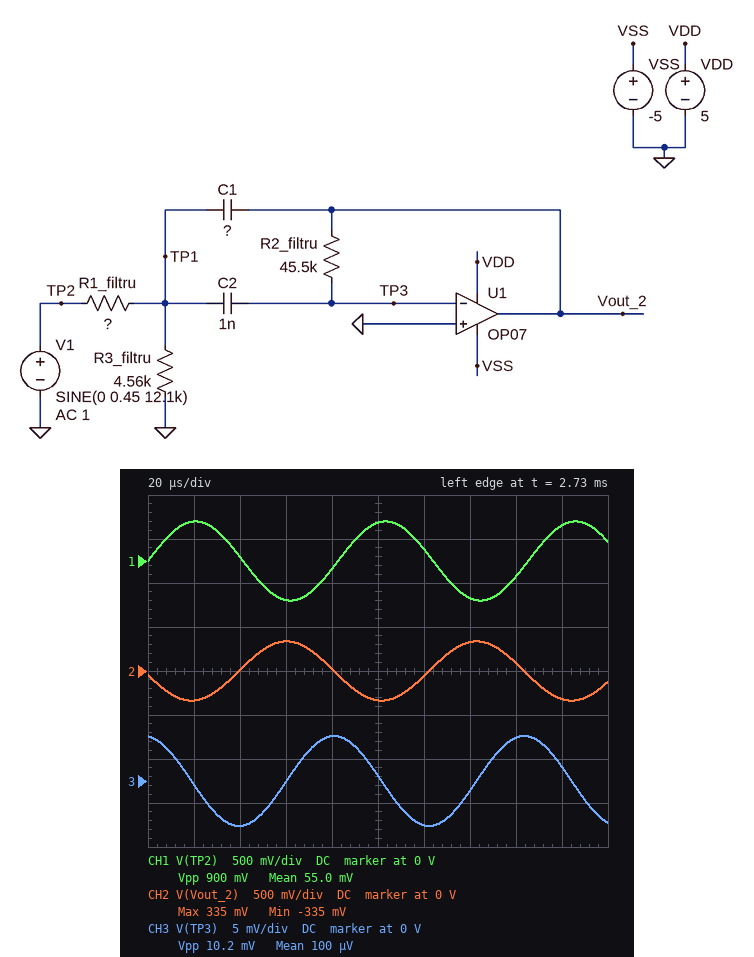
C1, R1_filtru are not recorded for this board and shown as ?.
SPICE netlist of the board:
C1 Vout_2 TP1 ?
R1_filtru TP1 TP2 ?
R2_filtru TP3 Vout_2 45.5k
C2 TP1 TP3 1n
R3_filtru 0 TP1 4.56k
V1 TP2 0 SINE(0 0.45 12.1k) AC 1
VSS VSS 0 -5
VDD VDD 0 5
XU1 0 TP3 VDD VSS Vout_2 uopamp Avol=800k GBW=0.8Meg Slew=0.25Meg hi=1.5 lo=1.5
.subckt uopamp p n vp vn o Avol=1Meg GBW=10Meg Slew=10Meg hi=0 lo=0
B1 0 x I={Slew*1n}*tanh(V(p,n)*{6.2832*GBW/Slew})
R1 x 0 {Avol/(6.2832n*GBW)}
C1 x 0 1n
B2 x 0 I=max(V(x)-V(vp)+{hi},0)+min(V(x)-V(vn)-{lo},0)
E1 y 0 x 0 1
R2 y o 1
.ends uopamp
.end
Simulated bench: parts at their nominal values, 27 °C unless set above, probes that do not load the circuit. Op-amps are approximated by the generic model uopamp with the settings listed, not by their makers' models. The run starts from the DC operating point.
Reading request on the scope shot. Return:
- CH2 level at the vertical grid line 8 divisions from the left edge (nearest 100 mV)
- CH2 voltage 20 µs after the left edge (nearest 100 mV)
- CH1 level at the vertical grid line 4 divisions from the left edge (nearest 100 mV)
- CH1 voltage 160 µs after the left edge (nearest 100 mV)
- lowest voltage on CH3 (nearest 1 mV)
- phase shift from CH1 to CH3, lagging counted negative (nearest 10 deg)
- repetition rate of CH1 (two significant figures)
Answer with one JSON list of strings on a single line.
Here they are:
["100 mV", "-300 mV", "-100 mV", "-200 mV", "-5 mV", "100 deg", "12 kHz"]
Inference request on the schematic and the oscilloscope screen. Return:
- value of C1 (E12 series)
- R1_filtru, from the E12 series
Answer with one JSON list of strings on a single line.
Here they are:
["820 pF", "33 kΩ"]
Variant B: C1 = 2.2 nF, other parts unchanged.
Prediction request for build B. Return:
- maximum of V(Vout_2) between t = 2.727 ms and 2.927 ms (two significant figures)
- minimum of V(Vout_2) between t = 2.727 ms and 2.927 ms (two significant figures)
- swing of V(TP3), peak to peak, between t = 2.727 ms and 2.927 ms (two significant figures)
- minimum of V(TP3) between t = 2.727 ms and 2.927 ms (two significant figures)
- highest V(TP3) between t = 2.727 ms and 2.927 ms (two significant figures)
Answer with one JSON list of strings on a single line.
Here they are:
["110 mV", "-110 mV", "3.4 mV", "-1.7 mV", "1.7 mV"]
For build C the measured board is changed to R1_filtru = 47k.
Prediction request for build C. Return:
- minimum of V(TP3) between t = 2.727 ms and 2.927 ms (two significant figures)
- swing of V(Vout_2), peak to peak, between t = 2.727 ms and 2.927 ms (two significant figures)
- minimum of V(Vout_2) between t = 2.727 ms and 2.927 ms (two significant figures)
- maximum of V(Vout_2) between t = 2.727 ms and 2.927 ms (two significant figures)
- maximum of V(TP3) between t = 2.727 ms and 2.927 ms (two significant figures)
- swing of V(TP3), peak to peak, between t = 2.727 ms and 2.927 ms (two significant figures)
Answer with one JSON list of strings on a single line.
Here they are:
["-3.6 mV", "480 mV", "-240 mV", "240 mV", "3.6 mV", "7.2 mV"]
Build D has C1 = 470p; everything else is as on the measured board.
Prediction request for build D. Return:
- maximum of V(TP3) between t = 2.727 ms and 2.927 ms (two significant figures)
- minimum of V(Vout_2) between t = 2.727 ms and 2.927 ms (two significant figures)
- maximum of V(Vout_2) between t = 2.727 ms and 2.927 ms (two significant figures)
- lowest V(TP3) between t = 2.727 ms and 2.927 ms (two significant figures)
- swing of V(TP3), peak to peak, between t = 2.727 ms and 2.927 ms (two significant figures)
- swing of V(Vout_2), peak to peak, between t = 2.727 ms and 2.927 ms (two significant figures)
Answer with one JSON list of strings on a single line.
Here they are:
["4.5 mV", "-300 mV", "300 mV", "-4.5 mV", "9.0 mV", "590 mV"]
